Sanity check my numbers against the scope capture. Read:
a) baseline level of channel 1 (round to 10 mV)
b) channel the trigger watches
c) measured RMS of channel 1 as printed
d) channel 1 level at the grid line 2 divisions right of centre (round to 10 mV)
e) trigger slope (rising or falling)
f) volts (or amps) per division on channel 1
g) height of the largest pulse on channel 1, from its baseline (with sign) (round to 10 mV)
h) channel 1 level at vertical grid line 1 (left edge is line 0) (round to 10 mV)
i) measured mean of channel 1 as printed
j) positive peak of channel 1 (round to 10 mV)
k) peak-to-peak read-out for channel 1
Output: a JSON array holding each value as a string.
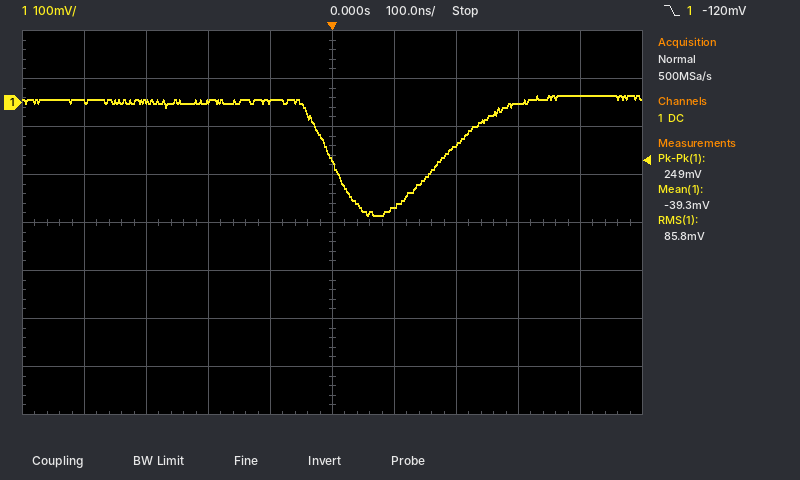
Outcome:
["0 mV", "channel 1", "85.8 mV", "-90 mV", "falling", "100 mV", "-240 mV", "0 mV", "-39.3 mV", "10 mV", "249 mV"]
